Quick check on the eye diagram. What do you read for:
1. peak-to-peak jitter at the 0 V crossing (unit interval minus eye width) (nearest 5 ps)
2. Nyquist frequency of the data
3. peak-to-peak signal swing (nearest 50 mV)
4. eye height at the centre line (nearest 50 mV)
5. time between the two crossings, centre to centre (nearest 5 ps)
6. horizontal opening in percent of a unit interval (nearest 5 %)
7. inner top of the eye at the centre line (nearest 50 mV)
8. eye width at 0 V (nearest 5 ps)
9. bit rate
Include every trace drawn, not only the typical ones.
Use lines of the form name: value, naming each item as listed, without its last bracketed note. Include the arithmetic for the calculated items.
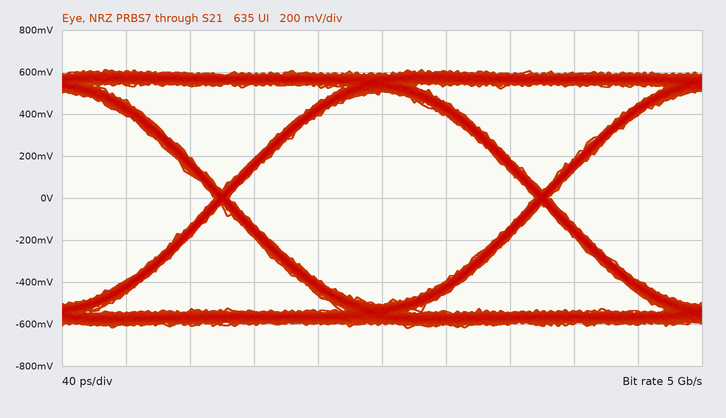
peak-to-peak jitter at the 0 V crossing (unit interval minus eye width): 10 ps
Nyquist frequency of the data: 2.5 GHz
peak-to-peak signal swing: 1.25 V
eye height at the centre line: 1.00 V
time between the two crossings, centre to centre: 200 ps
horizontal opening in percent of a unit interval: 190 ps / 200 ps ≈ 95 %
inner top of the eye at the centre line: 500 mV
eye width at 0 V: 190 ps
bit rate: 5 Gb/s
